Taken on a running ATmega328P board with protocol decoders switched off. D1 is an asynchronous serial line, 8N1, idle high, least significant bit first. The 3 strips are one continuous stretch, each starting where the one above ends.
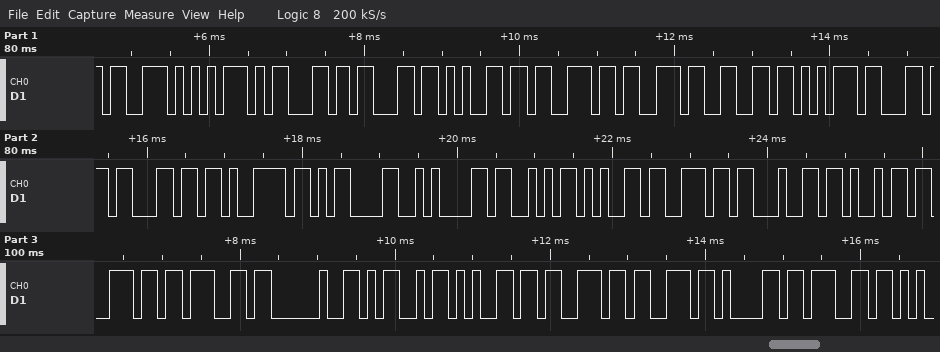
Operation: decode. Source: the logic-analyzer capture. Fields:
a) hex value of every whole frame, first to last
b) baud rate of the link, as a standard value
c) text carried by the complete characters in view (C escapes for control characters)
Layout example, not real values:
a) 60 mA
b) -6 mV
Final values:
a) 73 75 63 63 65 73 73 66 75 6C 6C 79 0D 0A 53 65 6E 64 69 6E 67 20 4D 65 73 73 61 67
b) 9600 baud
c) "successfully\r\nSending Messag"
